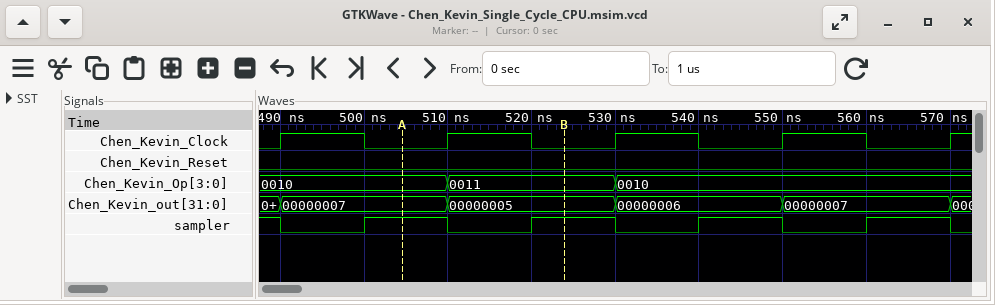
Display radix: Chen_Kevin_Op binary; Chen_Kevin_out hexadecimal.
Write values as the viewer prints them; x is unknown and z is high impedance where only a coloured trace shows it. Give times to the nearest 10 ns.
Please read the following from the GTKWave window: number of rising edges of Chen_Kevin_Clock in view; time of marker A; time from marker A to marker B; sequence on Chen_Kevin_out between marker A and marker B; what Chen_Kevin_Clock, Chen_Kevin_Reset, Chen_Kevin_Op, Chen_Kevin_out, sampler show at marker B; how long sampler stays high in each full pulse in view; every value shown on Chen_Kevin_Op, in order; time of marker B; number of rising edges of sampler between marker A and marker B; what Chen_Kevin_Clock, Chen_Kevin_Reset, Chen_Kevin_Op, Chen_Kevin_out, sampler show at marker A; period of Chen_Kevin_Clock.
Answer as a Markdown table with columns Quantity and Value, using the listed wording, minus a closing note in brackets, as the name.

| Quantity | Value |
|---|---|
| number of rising edges of Chen_Kevin_Clock in view | 5 |
| time of marker A | 500 ns |
| time from marker A to marker B | 20 ns |
| sequence on Chen_Kevin_out between marker A and marker B | 00000007, 00000005 |
| what Chen_Kevin_Clock, Chen_Kevin_Reset, Chen_Kevin_Op, Chen_Kevin_out, sampler show at marker B | Chen_Kevin_Clock=0, Chen_Kevin_Reset=0, Chen_Kevin_Op=0011, Chen_Kevin_out=00000005, sampler=1 |
| how long sampler stays high in each full pulse in view | 10 ns, 10 ns, 10 ns, 10 ns |
| every value shown on Chen_Kevin_Op, in order | 0010, 0011, 0010 |
| time of marker B | 520 ns |
| number of rising edges of sampler between marker A and marker B | 1 |
| what Chen_Kevin_Clock, Chen_Kevin_Reset, Chen_Kevin_Op, Chen_Kevin_out, sampler show at marker A | Chen_Kevin_Clock=0, Chen_Kevin_Reset=0, Chen_Kevin_Op=0010, Chen_Kevin_out=00000007, sampler=1 |
| period of Chen_Kevin_Clock | 20 ns |
